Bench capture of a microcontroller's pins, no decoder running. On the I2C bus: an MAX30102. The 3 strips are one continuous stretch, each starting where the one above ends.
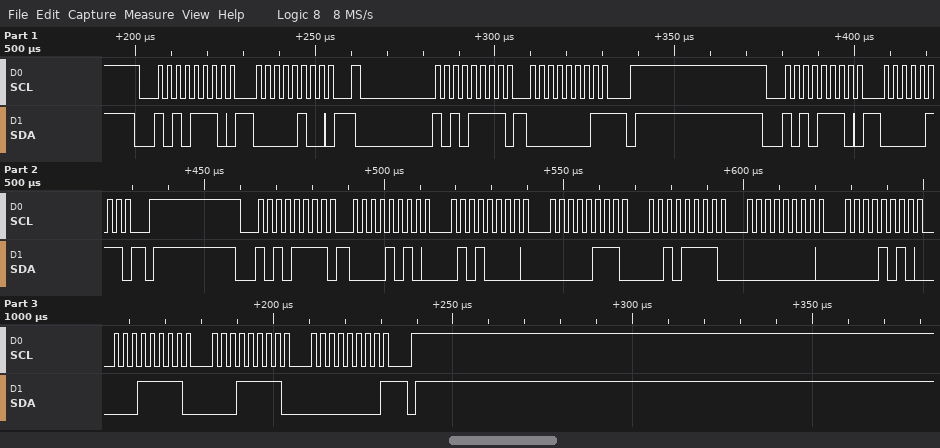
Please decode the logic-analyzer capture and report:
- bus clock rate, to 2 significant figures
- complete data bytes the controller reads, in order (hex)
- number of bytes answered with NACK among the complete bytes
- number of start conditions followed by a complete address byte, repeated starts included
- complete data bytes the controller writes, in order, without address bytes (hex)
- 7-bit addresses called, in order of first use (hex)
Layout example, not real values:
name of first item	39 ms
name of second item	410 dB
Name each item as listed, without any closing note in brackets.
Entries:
bus clock rate, to 2 significant figures	400 kHz
complete data bytes the controller reads, in order	01 0A 50 07 2F 00 0A 1F 1F 00
number of bytes answered with NACK among the complete bytes	2
number of start conditions followed by a complete address byte, repeated starts included	4
complete data bytes the controller writes, in order, without address bytes	04 07
7-bit addresses called, in order of first use	0x57
